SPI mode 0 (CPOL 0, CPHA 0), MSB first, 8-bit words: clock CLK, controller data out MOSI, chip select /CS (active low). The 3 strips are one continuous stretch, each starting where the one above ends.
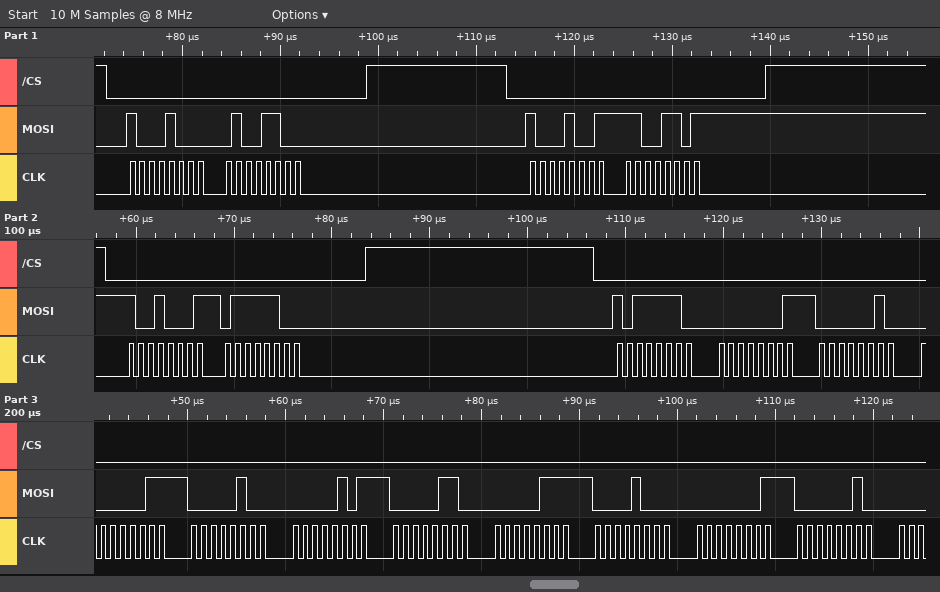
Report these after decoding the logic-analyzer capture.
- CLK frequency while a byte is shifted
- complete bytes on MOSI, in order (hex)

1 MHz
88 4C 89 CD 91 7C BE 01 02 03 04 05 06 07 08 01 02
